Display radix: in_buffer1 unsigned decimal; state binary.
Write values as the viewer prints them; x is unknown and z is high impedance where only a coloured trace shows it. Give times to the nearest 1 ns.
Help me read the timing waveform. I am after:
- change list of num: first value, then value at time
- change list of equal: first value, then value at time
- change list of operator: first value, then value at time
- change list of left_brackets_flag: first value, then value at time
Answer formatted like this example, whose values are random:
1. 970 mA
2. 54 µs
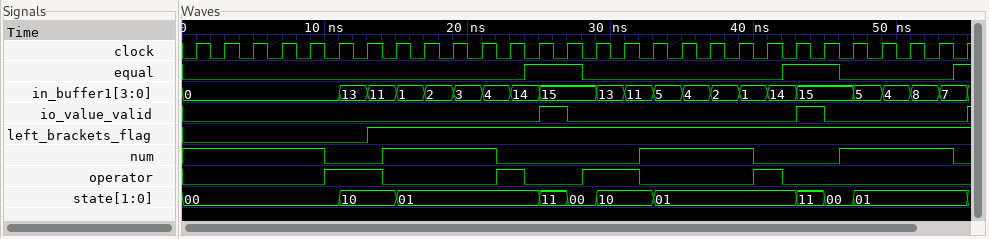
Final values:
1. 1, 0 at 10 ns, 1 at 14 ns, 0 at 22 ns, 1 at 32 ns, 0 at 40 ns, 1 at 46 ns, 0 at 54 ns
2. 0, 1 at 24 ns, 0 at 28 ns, 1 at 42 ns, 0 at 46 ns, 1 at 54 ns
3. 0, 1 at 10 ns, 0 at 14 ns, 1 at 22 ns, 0 at 24 ns, 1 at 28 ns, 0 at 32 ns, 1 at 40 ns, 0 at 42 ns
4. 0, 1 at 13 ns
